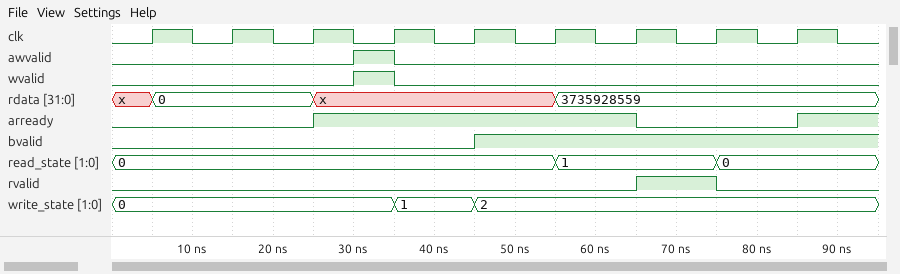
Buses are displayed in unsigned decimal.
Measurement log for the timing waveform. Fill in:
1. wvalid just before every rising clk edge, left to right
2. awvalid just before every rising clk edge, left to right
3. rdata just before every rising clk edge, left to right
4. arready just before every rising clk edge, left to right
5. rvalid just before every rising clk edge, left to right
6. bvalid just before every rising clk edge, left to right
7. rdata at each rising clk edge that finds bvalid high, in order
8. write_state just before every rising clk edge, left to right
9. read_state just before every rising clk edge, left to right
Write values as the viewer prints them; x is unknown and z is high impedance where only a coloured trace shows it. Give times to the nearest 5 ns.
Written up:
0 0 0 1 0 0 0 0 0
0 0 0 1 0 0 0 0 0
x, 0, 0, x, x, x, 3735928559, 3735928559, 3735928559
0 0 0 1 1 1 1 0 0
0 0 0 0 0 0 0 1 0
0 0 0 0 0 1 1 1 1
x, 3735928559, 3735928559, 3735928559
0, 0, 0, 0, 1, 2, 2, 2, 2
0, 0, 0, 0, 0, 0, 1, 1, 0
